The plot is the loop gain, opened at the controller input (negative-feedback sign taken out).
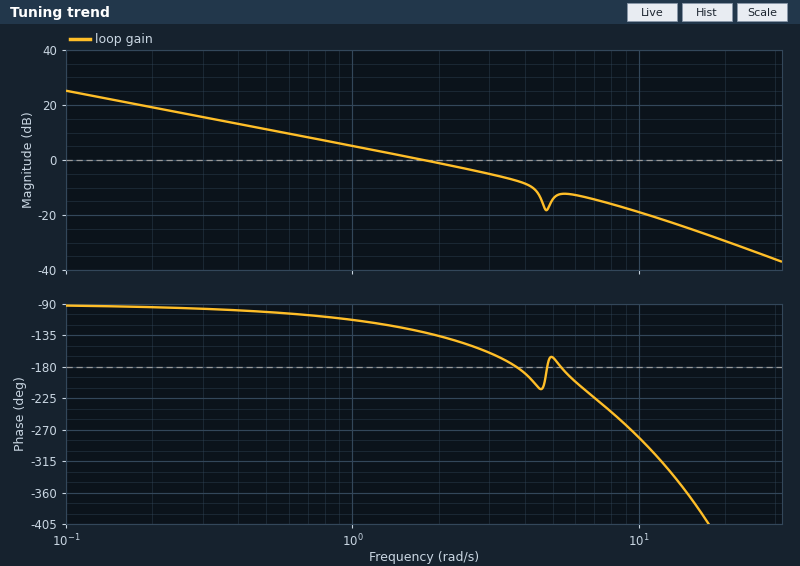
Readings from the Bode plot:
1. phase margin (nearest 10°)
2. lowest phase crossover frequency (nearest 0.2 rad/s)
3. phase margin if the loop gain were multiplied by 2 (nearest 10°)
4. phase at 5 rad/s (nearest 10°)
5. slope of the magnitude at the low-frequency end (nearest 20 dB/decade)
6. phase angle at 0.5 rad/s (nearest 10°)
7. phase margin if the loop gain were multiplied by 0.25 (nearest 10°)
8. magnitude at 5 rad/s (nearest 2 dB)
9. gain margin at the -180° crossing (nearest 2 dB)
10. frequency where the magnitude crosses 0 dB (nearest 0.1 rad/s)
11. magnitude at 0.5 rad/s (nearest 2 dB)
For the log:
50°
3.8 rad/s
10°
-170°
-20 dB/decade
-100°
80°
-14 dB
8 dB
1.8 rad/s
12 dB
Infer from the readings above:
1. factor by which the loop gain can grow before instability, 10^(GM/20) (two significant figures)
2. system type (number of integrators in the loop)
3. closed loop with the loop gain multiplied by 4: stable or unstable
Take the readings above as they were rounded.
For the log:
2.5
1
unstable
